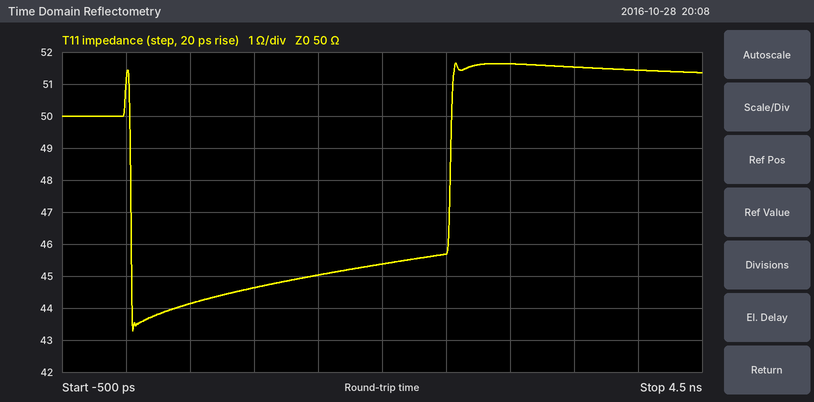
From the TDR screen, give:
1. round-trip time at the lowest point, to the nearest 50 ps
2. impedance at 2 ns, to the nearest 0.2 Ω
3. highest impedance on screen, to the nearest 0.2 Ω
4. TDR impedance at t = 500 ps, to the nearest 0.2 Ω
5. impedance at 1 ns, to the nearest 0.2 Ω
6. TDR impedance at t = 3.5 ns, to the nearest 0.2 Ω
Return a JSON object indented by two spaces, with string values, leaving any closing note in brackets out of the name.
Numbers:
{
  "round-trip time at the lowest point, to the nearest 50 ps": "50 ps",
  "impedance at 2 ns, to the nearest 0.2 Ω": "45.4 Ω",
  "highest impedance on screen, to the nearest 0.2 Ω": "51.6 Ω",
  "TDR impedance at t = 500 ps, to the nearest 0.2 Ω": "44.2 Ω",
  "impedance at 1 ns, to the nearest 0.2 Ω": "44.6 Ω",
  "TDR impedance at t = 3.5 ns, to the nearest 0.2 Ω": "51.6 Ω"
}
